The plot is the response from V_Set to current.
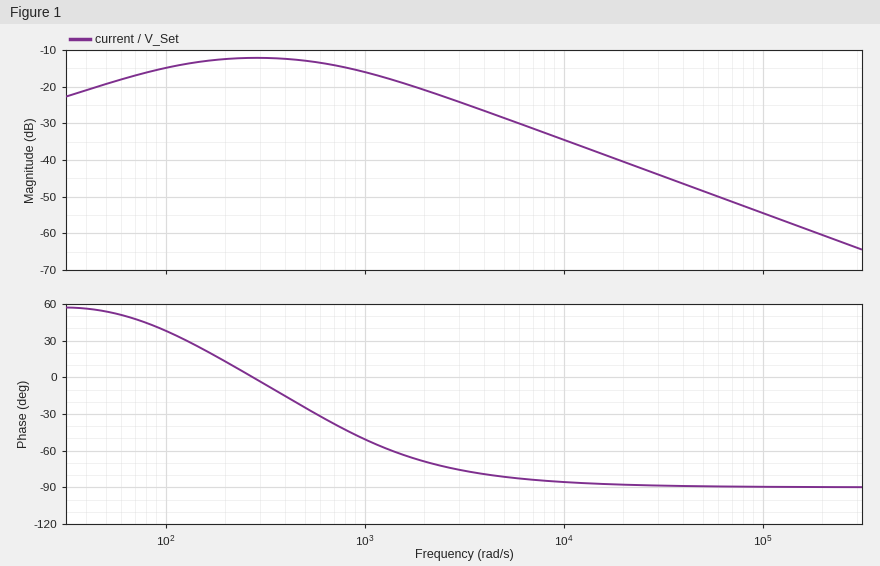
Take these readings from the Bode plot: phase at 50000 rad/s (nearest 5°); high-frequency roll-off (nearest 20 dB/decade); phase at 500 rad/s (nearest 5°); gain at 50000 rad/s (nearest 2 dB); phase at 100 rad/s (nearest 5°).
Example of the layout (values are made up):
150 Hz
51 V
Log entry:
-90°
-20 dB/decade
-25°
-48 dB
40°
